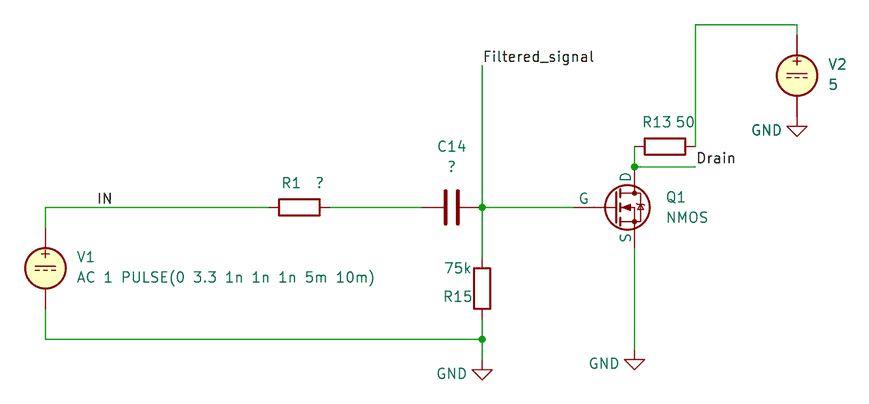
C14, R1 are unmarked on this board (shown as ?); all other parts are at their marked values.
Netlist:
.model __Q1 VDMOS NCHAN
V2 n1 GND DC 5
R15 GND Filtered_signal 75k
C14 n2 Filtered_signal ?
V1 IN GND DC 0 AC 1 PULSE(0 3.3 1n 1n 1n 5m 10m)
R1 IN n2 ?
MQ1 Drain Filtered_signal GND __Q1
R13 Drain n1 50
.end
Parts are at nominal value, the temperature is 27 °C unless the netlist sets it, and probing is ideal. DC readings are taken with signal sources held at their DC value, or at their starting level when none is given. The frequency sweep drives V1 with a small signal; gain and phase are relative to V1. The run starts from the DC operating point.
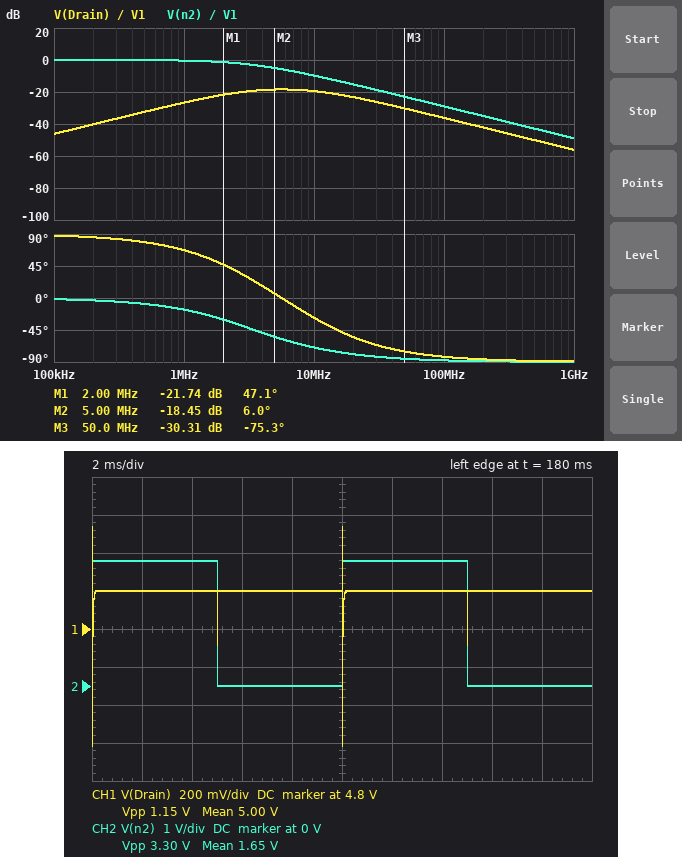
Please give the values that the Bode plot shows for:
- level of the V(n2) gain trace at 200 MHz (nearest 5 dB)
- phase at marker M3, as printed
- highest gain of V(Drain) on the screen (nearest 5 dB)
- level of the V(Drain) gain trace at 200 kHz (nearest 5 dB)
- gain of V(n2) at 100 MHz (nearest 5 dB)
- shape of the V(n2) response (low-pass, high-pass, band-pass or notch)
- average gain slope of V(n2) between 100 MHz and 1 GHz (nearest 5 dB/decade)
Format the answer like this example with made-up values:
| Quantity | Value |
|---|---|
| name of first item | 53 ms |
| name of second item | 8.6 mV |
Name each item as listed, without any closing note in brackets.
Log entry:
| Quantity | Value |
|---|---|
| level of the V(n2) gain trace at 200 MHz | -35 dB |
| phase at marker M3, as printed | -75.3 deg |
| highest gain of V(Drain) on the screen | -20 dB |
| level of the V(Drain) gain trace at 200 kHz | -40 dB |
| gain of V(n2) at 100 MHz | -30 dB |
| shape of the V(n2) response | low-pass |
| average gain slope of V(n2) between 100 MHz and 1 GHz | -20 dB/decade |
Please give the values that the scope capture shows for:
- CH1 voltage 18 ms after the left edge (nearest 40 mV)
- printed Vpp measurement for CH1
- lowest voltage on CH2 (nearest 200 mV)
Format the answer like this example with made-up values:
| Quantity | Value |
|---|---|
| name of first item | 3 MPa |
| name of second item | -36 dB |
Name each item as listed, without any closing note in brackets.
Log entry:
| Quantity | Value |
|---|---|
| CH1 voltage 18 ms after the left edge | 5.00 V |
| printed Vpp measurement for CH1 | 1.15 V |
| lowest voltage on CH2 | 0 V |
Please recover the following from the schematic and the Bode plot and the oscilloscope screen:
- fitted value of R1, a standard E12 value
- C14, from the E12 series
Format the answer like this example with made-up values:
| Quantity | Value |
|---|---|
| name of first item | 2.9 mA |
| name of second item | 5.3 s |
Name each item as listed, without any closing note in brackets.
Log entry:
| Quantity | Value |
|---|---|
| fitted value of R1, a standard E12 value | 33 Ω |
| C14, from the E12 series | 15 nF |
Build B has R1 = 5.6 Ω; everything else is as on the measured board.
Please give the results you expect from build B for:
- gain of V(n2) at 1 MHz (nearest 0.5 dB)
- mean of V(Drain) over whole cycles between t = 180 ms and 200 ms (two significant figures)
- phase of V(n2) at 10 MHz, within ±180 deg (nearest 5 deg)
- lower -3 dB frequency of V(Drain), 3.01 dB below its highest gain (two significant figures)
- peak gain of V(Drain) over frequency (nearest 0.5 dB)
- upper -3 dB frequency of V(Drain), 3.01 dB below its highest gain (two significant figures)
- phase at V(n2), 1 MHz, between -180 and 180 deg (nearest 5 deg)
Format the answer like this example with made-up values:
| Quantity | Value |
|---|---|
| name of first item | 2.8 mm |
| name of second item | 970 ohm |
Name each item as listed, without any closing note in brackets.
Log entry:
| Quantity | Value |
|---|---|
| gain of V(n2) at 1 MHz | 0 dB |
| mean of V(Drain) over whole cycles between t = 180 ms and 200 ms | 5.0 V |
| phase of V(n2) at 10 MHz, within ±180 deg | -25 deg |
| lower -3 dB frequency of V(Drain), 3.01 dB below its highest gain | 5.3 MHz |
| peak gain of V(Drain) over frequency | -10.5 dB |
| upper -3 dB frequency of V(Drain), 3.01 dB below its highest gain | 36 MHz |
| phase at V(n2), 1 MHz, between -180 and 180 deg | -5 deg |
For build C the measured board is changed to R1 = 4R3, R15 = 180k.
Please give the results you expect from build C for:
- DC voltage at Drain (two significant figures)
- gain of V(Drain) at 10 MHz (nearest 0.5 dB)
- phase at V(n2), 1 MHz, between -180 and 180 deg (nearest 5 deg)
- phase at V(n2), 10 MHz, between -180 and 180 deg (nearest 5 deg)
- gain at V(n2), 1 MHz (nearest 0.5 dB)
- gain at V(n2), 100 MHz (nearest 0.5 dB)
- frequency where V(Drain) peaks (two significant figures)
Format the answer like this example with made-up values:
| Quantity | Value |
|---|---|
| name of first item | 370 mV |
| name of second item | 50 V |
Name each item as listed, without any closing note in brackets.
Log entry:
| Quantity | Value |
|---|---|
| DC voltage at Drain | 5.0 V |
| gain of V(Drain) at 10 MHz | -10.5 dB |
| phase at V(n2), 1 MHz, between -180 and 180 deg | 0 deg |
| phase at V(n2), 10 MHz, between -180 and 180 deg | -20 deg |
| gain at V(n2), 1 MHz | 0 dB |
| gain at V(n2), 100 MHz | -11.5 dB |
| frequency where V(Drain) peaks | 16 MHz |
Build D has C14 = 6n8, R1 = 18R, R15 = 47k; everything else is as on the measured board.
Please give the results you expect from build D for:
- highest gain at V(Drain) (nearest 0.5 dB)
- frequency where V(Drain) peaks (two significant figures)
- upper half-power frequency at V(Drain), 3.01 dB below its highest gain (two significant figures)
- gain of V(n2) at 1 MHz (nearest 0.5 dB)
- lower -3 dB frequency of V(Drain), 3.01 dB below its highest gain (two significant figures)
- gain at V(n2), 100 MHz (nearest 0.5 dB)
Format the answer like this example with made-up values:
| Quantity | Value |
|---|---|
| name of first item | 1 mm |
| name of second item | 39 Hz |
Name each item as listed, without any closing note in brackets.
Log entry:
| Quantity | Value |
|---|---|
| highest gain at V(Drain) | -15.5 dB |
| frequency where V(Drain) peaks | 8.1 MHz |
| upper half-power frequency at V(Drain), 3.01 dB below its highest gain | 20 MHz |
| gain of V(n2) at 1 MHz | 0 dB |
| lower -3 dB frequency of V(Drain), 3.01 dB below its highest gain | 3.3 MHz |
| gain at V(n2), 100 MHz | -23.0 dB |
